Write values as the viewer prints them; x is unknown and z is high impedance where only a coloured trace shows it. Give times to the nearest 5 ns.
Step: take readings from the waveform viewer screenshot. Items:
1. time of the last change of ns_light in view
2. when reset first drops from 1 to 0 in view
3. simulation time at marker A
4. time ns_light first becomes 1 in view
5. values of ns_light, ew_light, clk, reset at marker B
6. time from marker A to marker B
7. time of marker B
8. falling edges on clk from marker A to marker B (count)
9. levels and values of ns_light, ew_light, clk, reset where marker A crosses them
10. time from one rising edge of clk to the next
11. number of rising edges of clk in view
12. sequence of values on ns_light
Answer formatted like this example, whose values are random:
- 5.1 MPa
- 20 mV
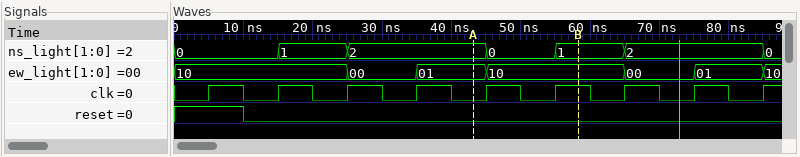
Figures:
- 85 ns
- 10 ns
- 45 ns
- 15 ns
- ns_light=1, ew_light=10, clk=1, reset=0
- 15 ns
- 60 ns
- 1
- ns_light=2, ew_light=01, clk=0, reset=0
- 10 ns
- 9
- 0, 1, 2, 0, 1, 2, 0
